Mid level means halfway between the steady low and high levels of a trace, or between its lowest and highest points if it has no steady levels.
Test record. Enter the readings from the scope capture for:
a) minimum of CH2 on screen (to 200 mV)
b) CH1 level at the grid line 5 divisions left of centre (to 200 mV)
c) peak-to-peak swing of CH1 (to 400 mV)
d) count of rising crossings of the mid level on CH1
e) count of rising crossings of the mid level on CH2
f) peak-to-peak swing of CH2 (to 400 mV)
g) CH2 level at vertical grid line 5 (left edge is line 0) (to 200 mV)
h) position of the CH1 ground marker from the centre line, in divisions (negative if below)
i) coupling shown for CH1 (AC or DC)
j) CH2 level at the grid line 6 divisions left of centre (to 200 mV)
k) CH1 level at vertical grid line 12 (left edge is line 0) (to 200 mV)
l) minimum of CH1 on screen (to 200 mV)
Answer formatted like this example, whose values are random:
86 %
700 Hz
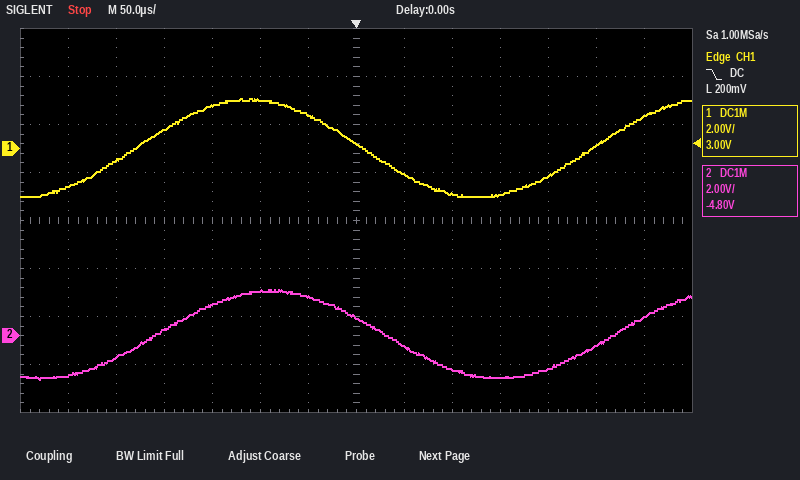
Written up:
-1.8 V
-400 mV
4.0 V
2
2
3.6 V
1.8 V
+1.5 div
DC
-1.6 V
200 mV
-2.0 V
